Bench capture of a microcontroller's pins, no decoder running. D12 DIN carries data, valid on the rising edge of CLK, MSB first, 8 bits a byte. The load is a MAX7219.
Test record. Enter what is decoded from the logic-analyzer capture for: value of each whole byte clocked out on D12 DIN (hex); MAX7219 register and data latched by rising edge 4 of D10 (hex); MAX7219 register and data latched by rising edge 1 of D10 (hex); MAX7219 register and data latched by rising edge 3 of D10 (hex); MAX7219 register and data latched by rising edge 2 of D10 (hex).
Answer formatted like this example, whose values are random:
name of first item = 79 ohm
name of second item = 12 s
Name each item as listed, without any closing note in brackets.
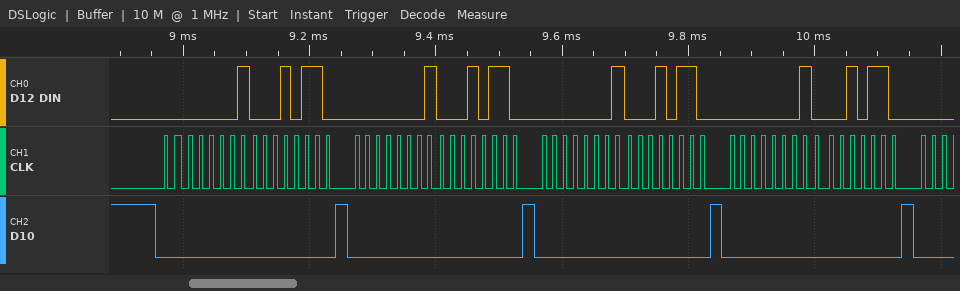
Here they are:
value of each whole byte clocked out on D12 DIN = 01 16 01 16 01 16 01 16
MAX7219 register and data latched by rising edge 4 of D10 = register 0x1, data 0x16
MAX7219 register and data latched by rising edge 1 of D10 = register 0x1, data 0x16
MAX7219 register and data latched by rising edge 3 of D10 = register 0x1, data 0x16
MAX7219 register and data latched by rising edge 2 of D10 = register 0x1, data 0x16
